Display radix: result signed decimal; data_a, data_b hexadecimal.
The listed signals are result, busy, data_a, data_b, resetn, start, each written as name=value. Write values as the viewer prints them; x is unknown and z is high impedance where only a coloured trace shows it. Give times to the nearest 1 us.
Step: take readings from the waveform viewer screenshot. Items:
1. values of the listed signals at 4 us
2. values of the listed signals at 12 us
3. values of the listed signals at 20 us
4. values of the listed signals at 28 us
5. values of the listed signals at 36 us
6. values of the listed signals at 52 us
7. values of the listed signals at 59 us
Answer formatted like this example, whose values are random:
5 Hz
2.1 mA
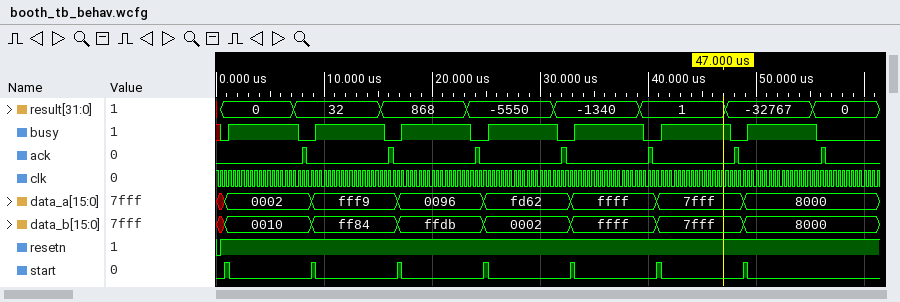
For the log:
result=0, busy=1, data_a=0002, data_b=0010, resetn=1, start=0
result=32, busy=1, data_a=fff9, data_b=ff84, resetn=1, start=0
result=868, busy=1, data_a=0096, data_b=ffdb, resetn=1, start=0
result=-5550, busy=1, data_a=fd62, data_b=0002, resetn=1, start=0
result=-1340, busy=1, data_a=ffff, data_b=ffff, resetn=1, start=0
result=-32767, busy=1, data_a=8000, data_b=8000, resetn=1, start=0
result=0, busy=0, data_a=8000, data_b=8000, resetn=1, start=0
